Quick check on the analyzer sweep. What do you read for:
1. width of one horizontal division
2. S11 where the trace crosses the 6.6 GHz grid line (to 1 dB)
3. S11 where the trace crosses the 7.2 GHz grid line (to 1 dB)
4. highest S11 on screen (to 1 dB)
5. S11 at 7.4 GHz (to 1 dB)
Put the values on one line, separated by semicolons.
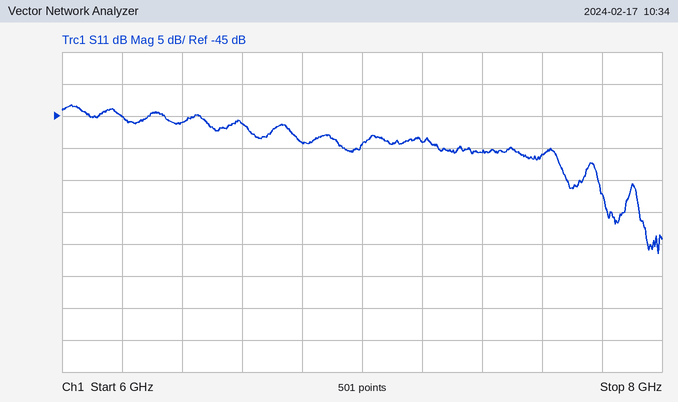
200 MHz; -46 dB; -49 dB; -43 dB; -51 dB
